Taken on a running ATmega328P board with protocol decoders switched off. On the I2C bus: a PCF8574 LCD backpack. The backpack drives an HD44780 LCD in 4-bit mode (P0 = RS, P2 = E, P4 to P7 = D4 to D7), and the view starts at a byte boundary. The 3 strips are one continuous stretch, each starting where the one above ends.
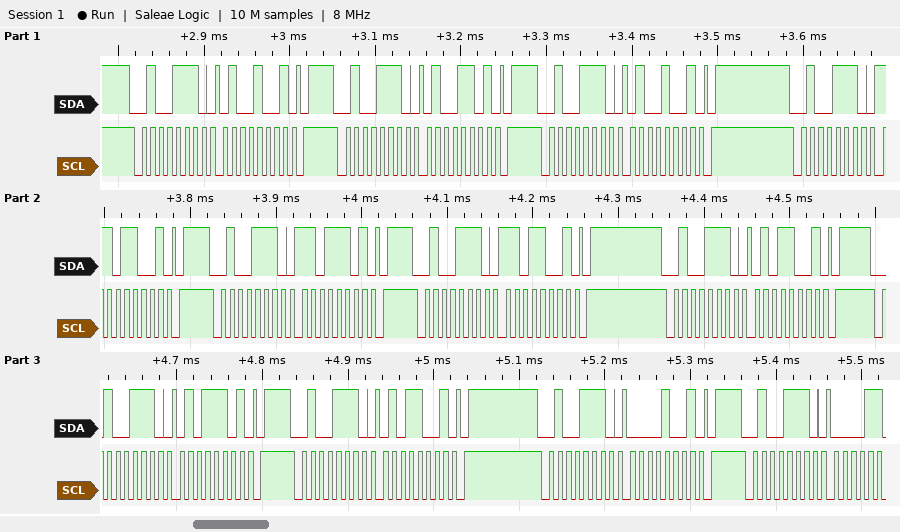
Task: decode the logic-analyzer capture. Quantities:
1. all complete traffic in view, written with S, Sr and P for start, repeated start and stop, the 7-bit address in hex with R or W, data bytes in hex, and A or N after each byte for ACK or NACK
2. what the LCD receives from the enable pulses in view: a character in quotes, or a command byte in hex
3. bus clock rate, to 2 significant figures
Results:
S 27W A 49 A P S 27W A 4D A P S 27W A 49 A P S 27W A D9 A P S 27W A DD A P S 27W A D9 A P S 27W A 59 A P S 27W A 5D A P S 27W A 59 A P S 27W A 09 A P S 27W A
'M'
100 kHz
